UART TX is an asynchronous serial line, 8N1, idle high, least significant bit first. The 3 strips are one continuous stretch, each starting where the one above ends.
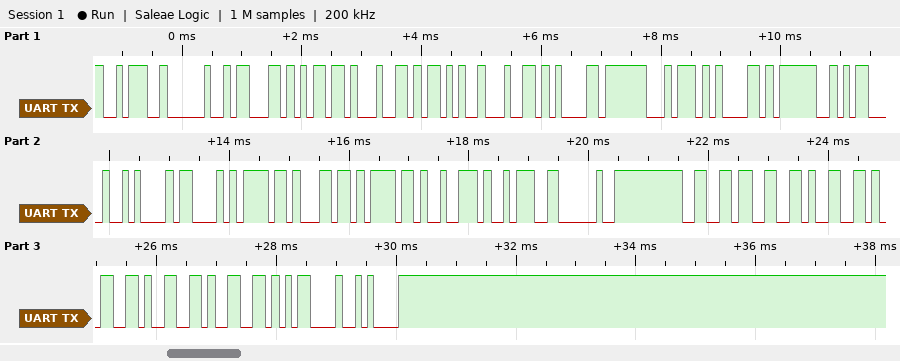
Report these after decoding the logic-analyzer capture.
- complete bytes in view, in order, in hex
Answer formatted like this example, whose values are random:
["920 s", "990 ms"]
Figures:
["0x3A 0x20 0x63 0x6D 0x64 0x2B 0x64 0x61 0x74 0x61 0x3F 0x0D 0x0A 0x43 0x6F 0x6C 0x6F 0x72 0x3A 0x20 0x66 0x66 0x66 0x66 0x66 0x66 0x0D 0x0A"]
